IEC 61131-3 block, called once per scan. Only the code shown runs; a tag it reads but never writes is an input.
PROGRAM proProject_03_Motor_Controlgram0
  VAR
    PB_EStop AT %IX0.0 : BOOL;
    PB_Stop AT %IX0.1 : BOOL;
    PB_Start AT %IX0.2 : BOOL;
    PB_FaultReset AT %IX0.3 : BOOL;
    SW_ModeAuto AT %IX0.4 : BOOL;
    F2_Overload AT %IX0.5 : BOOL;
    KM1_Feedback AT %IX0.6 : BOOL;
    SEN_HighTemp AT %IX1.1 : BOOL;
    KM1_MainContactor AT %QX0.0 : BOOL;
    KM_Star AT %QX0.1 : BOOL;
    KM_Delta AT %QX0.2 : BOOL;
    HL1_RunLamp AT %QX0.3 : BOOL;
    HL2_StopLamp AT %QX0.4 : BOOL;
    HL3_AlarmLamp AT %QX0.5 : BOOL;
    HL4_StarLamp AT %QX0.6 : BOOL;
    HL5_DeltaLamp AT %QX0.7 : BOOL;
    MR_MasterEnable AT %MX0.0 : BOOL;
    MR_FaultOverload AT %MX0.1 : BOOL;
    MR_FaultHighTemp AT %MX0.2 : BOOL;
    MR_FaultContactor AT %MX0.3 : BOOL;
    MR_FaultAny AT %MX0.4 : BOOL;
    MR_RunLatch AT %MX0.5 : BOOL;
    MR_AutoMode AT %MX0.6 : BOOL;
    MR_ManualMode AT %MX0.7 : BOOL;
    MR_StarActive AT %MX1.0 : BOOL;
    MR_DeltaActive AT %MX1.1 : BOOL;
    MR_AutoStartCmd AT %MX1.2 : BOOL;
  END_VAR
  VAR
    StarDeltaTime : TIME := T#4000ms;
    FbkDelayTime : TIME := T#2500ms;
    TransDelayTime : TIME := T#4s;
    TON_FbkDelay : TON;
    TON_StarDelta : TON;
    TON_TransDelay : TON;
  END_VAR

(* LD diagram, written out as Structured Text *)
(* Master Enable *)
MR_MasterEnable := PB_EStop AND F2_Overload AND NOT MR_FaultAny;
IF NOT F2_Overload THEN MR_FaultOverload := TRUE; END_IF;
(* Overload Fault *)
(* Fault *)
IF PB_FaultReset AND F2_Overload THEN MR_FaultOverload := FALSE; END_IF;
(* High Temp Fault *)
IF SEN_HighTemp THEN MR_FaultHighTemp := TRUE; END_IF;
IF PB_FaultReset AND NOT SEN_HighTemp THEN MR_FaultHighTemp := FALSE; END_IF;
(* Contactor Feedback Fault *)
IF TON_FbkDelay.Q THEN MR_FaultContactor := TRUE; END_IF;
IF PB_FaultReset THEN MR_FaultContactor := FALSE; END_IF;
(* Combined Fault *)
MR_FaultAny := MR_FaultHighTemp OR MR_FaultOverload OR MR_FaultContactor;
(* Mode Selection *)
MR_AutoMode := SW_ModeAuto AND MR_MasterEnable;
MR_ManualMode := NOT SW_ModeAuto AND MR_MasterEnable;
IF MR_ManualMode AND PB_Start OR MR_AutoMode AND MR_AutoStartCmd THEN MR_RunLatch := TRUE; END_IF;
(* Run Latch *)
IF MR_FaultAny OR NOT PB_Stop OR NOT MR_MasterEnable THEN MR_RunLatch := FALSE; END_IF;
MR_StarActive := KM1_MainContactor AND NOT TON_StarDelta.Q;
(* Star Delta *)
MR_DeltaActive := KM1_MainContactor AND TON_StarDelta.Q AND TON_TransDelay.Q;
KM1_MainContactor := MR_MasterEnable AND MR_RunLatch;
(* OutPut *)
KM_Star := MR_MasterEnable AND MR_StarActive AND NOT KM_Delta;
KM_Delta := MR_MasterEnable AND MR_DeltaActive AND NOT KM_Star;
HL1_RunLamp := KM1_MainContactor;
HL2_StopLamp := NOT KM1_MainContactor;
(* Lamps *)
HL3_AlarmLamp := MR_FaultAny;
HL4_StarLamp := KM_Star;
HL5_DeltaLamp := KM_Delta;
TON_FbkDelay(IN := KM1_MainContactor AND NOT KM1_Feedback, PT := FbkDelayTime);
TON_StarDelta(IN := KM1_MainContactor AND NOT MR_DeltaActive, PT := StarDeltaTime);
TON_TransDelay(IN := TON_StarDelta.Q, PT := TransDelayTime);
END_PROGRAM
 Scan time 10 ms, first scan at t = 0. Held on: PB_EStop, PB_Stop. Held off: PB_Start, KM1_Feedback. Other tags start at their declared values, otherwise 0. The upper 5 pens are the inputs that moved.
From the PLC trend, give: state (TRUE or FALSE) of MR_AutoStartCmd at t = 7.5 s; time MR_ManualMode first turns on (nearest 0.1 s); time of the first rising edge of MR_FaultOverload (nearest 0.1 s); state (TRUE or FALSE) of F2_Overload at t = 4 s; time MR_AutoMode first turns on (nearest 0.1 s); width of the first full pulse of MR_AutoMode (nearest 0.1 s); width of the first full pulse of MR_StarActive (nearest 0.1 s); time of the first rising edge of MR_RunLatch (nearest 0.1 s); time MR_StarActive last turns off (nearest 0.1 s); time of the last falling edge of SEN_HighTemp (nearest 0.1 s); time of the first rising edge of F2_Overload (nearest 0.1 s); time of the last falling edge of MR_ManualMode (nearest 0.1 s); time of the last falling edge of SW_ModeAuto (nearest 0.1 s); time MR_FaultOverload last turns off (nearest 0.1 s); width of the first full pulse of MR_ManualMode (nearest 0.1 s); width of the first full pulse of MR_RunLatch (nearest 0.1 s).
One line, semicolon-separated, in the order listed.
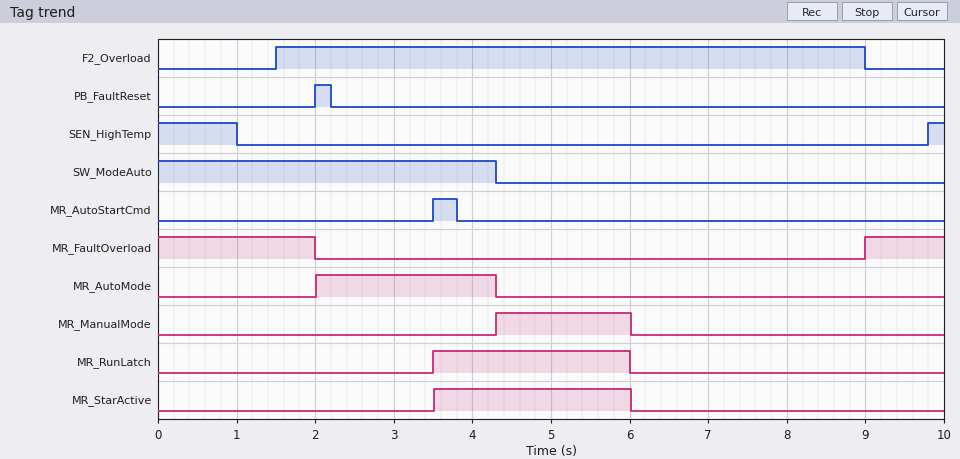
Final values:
FALSE; 4.3 s; 9.0 s; TRUE; 2.0 s; 2.3 s; 2.5 s; 3.5 s; 6.0 s; 1.0 s; 1.5 s; 6.0 s; 4.3 s; 2.0 s; 1.7 s; 2.5 s
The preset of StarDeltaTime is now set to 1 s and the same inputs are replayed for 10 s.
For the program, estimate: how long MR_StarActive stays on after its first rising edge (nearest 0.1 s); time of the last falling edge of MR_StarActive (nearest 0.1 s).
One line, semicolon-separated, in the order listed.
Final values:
1.0 s; 4.5 s
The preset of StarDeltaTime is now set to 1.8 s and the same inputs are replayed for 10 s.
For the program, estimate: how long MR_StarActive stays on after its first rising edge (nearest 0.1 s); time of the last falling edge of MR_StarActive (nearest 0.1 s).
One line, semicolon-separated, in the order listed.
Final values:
1.8 s; 5.3 s
